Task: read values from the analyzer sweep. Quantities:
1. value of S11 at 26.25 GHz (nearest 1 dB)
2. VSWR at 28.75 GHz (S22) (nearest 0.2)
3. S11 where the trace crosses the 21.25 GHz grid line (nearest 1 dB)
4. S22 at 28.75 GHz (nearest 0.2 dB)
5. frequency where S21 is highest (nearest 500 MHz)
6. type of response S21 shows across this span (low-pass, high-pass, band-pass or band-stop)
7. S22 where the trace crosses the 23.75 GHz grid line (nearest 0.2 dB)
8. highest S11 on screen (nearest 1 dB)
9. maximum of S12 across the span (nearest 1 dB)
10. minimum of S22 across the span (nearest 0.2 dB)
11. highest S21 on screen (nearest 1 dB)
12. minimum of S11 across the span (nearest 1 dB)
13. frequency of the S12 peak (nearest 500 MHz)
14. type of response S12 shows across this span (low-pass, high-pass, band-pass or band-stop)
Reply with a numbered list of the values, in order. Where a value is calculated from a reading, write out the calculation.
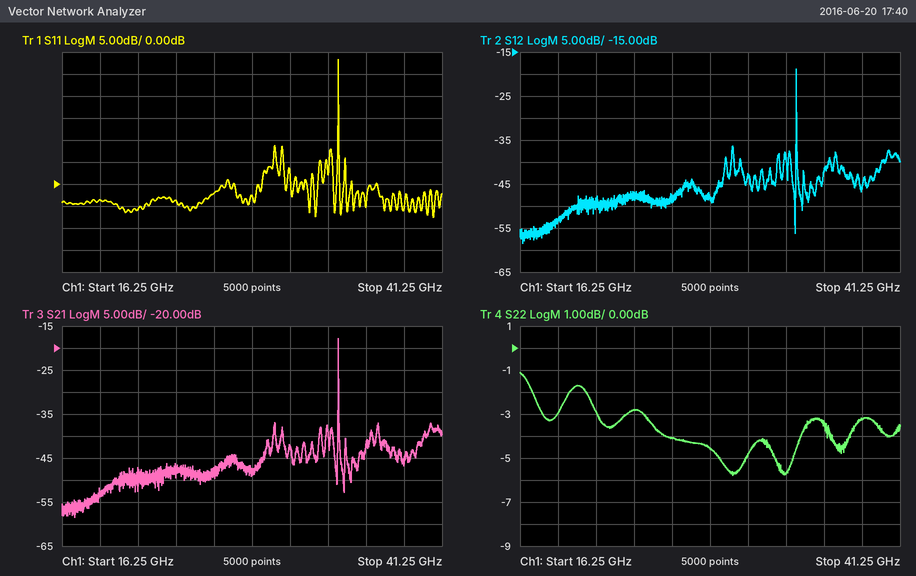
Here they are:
1. -2 dB
2. |Γ| = 10^(-4.6/20) = 0.5888; VSWR = (1 + 0.5888)/(1 − 0.5888) ≈ 3.86, so 3.8 to the nearest 0.2
3. -6 dB
4. -4.6 dB
5. 34.5 GHz
6. band-pass
7. -2.8 dB
8. 28 dB
9. -19 dB
10. -5.8 dB
11. -18 dB
12. -8 dB
13. 34.5 GHz
14. band-pass
